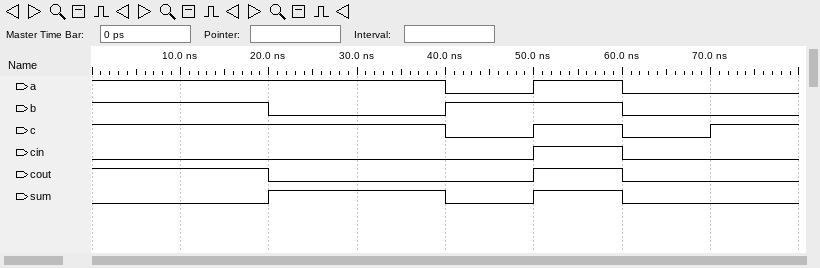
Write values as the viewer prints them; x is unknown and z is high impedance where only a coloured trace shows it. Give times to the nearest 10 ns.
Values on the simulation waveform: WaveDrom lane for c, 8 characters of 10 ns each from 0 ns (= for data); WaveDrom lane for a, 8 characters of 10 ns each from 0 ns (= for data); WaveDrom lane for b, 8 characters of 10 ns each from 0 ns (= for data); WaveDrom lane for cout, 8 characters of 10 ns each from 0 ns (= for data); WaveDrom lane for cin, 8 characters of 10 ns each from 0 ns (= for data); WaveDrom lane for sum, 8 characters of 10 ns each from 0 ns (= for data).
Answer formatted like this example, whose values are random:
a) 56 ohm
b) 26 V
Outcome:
a) {name: 'c', wave: '1...0101'}
b) {name: 'a', wave: '1...010.'}
c) {name: 'b', wave: '1.0.1.0.'}
d) {name: 'cout', wave: '1.0..10.'}
e) {name: 'cin', wave: '0....10.'}
f) {name: 'sum', wave: '0.1.010.'}
